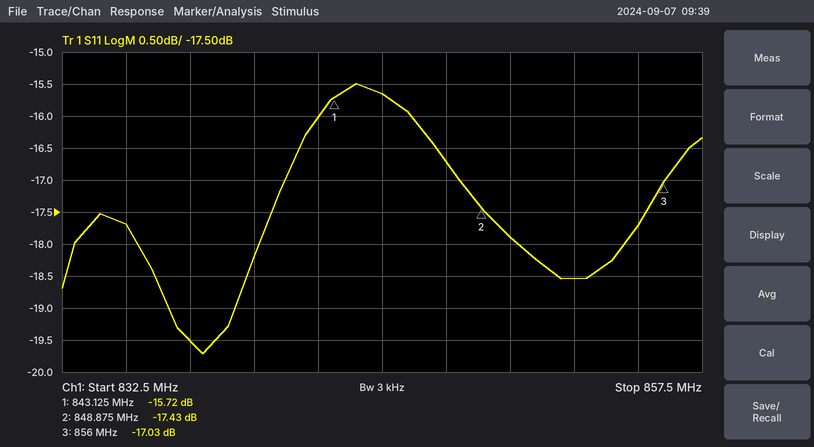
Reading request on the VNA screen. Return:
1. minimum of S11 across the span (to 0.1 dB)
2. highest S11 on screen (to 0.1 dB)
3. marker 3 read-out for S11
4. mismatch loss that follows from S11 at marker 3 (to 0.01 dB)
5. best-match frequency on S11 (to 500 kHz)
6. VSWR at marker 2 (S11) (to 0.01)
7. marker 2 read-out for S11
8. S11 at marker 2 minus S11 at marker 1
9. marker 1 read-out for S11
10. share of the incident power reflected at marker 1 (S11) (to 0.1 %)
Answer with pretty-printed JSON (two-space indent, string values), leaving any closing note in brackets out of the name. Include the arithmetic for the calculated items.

{
  "minimum of S11 across the span": "-19.7 dB",
  "highest S11 on screen": "-15.5 dB",
  "marker 3 read-out for S11": "-17.03 dB",
  "mismatch loss that follows from S11 at marker 3": "−10 log10(1 − 10^(-17.03/10)) ≈ 0.09 dB",
  "best-match frequency on S11": "838.0 MHz",
  "VSWR at marker 2 (S11)": "(1 + 0.1344)/(1 − 0.1344) ≈ 1.31",
  "marker 2 read-out for S11": "-17.43 dB",
  "S11 at marker 2 minus S11 at marker 1": "-17.43 − (-15.72) = -1.71 dB",
  "marker 1 read-out for S11": "-15.72 dB",
  "share of the incident power reflected at marker 1 (S11)": "10^(-15.72/10) ≈ 2.7 %"
}
